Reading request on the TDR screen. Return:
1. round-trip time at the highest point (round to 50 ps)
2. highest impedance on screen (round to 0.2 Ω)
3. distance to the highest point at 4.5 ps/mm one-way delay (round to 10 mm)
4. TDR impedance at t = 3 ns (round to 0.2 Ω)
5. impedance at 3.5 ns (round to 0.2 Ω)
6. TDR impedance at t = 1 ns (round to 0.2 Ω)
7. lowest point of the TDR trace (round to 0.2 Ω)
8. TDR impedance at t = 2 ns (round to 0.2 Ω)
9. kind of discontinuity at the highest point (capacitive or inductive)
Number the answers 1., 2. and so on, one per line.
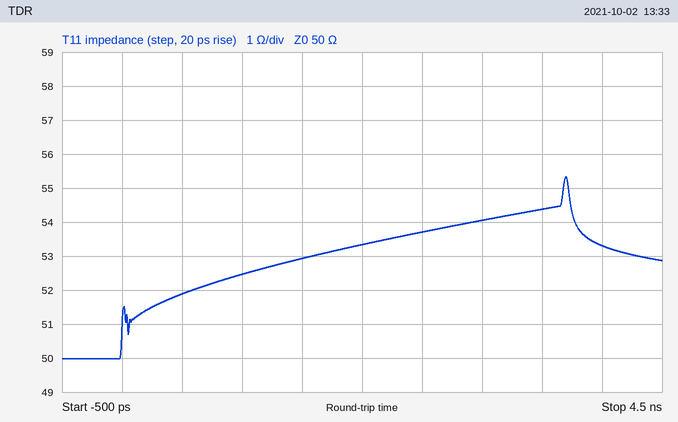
1. 3.70 ns
2. 55.4 Ω
3. 410 mm
4. 54.0 Ω
5. 54.4 Ω
6. 52.4 Ω
7. 50.0 Ω
8. 53.4 Ω
9. inductive
